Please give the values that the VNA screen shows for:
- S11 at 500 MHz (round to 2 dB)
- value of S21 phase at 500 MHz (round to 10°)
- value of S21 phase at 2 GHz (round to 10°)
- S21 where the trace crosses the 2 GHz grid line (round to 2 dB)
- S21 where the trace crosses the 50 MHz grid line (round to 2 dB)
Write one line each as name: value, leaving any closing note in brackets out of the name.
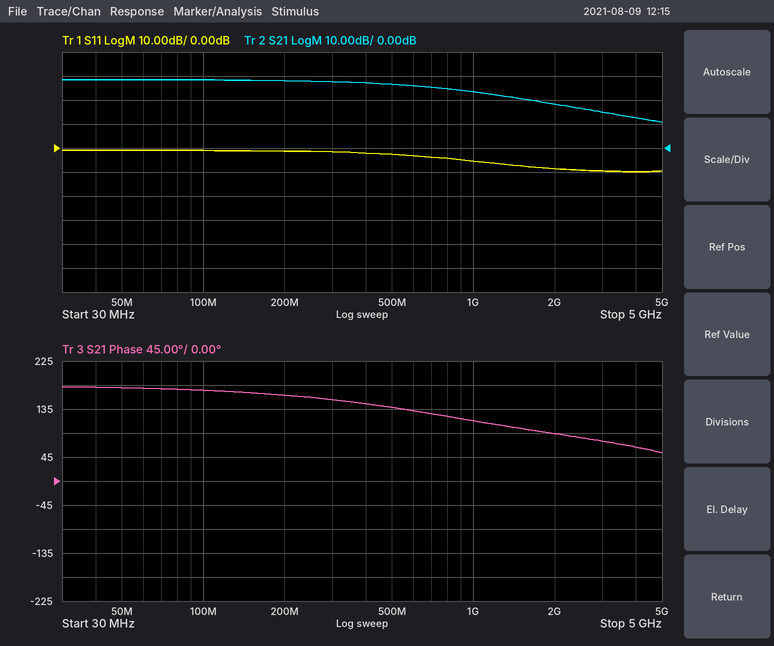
S11 at 500 MHz: -2 dB
value of S21 phase at 500 MHz: 140°
value of S21 phase at 2 GHz: 90°
S21 where the trace crosses the 2 GHz grid line: 18 dB
S21 where the trace crosses the 50 MHz grid line: 28 dB
